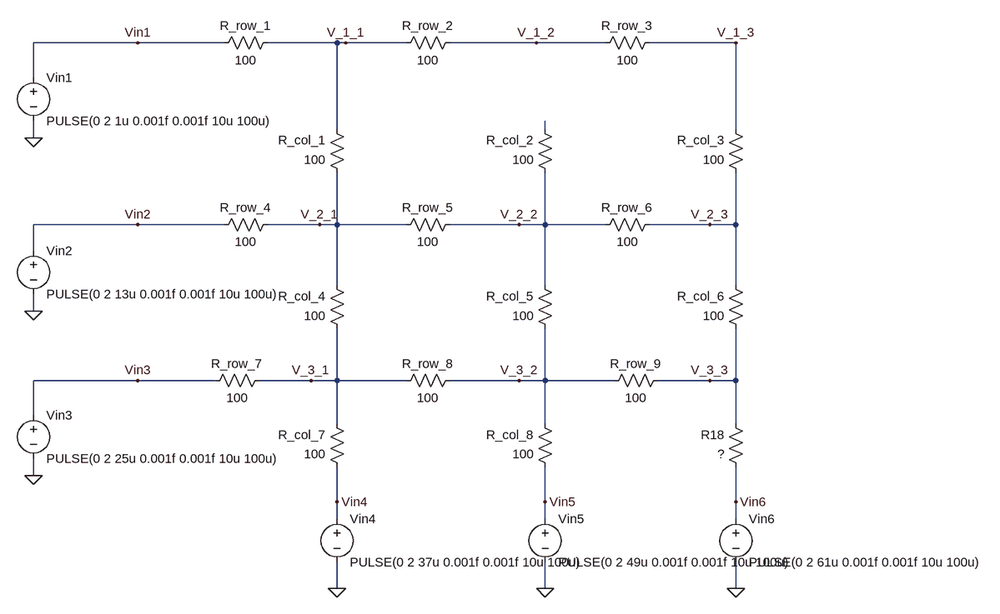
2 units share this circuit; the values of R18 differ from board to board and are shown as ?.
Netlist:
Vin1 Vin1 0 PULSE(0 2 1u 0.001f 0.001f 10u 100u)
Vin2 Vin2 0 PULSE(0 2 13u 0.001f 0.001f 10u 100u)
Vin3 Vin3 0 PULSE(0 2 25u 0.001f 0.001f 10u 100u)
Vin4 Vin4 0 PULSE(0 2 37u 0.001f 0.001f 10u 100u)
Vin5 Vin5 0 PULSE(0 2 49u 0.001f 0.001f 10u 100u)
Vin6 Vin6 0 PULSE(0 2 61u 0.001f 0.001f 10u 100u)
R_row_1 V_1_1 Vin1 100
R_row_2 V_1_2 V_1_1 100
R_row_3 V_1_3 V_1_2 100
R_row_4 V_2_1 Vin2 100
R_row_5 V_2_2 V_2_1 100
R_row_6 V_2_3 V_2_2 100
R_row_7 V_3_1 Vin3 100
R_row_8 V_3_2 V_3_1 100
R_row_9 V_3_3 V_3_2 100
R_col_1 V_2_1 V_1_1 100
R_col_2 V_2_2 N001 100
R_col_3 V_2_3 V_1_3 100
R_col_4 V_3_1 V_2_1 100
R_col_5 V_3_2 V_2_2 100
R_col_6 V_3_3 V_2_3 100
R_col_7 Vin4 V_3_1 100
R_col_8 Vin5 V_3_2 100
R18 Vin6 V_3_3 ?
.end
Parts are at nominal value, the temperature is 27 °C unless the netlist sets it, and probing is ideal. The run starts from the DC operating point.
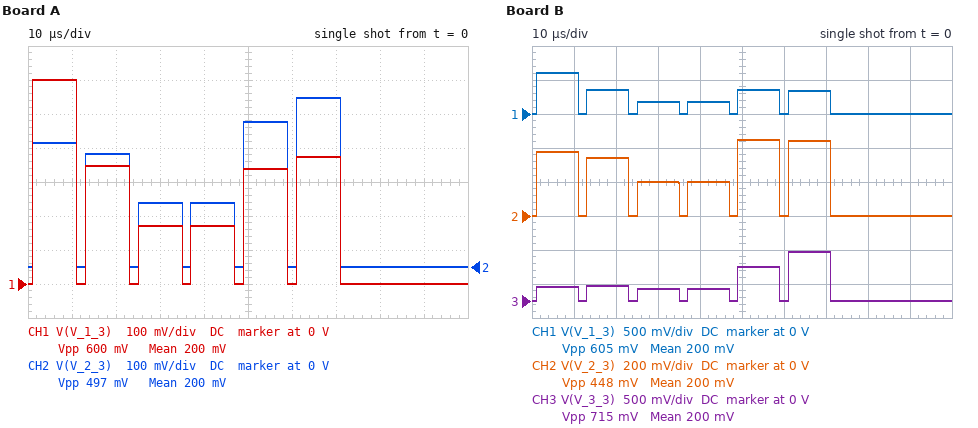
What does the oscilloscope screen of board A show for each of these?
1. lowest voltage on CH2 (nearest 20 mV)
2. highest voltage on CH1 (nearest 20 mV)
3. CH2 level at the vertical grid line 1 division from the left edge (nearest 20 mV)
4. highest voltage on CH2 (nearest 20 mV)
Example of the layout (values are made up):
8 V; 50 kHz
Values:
0 V; 600 mV; 360 mV; 500 mV
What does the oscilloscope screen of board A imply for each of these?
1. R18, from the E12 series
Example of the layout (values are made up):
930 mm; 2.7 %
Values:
150 Ω
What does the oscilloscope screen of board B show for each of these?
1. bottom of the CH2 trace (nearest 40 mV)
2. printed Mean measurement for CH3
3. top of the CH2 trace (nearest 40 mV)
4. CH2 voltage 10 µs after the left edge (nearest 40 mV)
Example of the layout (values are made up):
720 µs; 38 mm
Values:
0 V; 200 mV; 440 mV; 360 mV
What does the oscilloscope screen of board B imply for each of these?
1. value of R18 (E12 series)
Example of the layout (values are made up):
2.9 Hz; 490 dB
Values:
180 Ω
